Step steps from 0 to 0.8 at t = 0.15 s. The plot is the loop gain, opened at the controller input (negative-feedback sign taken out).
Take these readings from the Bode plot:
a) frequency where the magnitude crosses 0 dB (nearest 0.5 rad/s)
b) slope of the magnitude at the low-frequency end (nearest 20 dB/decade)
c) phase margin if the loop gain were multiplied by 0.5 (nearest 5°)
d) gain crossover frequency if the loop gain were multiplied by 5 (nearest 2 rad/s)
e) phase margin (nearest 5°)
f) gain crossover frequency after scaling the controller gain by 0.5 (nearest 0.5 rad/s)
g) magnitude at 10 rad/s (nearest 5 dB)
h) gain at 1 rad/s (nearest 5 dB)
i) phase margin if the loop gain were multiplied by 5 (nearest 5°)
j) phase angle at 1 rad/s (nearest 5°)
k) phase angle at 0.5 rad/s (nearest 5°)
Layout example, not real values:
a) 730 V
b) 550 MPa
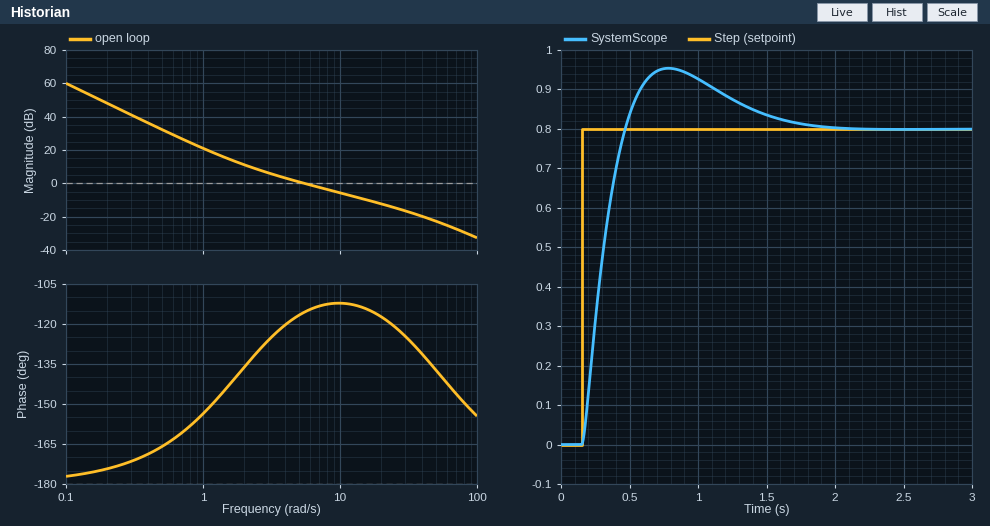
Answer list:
a) 5.5 rad/s
b) -40 dB/decade
c) 55°
d) 24 rad/s
e) 65°
f) 3.0 rad/s
g) -5 dB
h) 20 dB
i) 60°
j) -155°
k) -165°
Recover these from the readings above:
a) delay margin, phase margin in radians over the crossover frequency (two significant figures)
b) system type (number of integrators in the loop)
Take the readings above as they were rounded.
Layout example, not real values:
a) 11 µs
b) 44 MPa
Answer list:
a) 0.21 s
b) 2
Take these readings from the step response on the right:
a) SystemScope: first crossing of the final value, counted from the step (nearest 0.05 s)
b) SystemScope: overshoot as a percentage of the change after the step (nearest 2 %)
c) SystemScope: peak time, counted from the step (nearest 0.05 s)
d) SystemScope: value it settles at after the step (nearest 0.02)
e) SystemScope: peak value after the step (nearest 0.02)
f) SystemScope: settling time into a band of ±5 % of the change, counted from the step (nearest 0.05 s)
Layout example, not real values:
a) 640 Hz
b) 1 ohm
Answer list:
a) 0.30 s
b) 20 %
c) 0.65 s
d) 0.80
e) 0.96
f) 1.30 s
